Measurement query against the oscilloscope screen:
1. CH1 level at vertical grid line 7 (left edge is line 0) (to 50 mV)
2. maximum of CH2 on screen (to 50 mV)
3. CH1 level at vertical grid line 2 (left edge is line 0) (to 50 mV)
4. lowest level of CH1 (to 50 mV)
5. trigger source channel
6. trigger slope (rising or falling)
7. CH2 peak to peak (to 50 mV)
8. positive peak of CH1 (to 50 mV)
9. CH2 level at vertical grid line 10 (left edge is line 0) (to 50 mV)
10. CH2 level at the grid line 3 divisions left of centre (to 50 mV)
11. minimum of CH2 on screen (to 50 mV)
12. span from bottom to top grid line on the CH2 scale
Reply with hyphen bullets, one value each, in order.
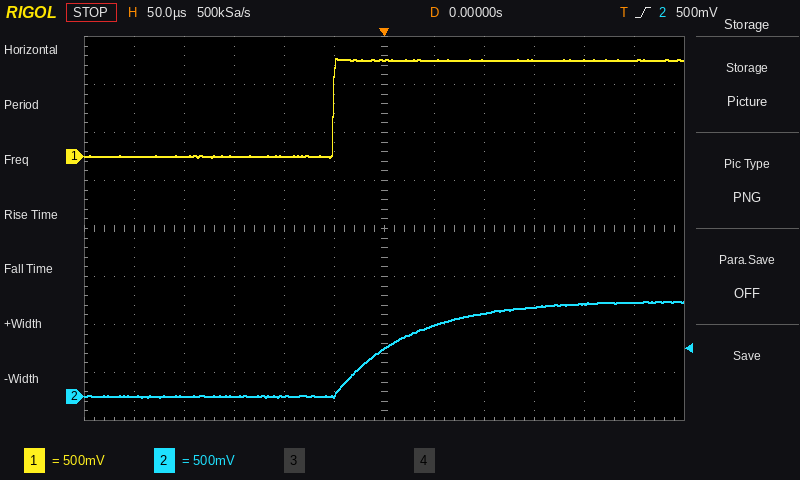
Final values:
- 1.00 V
- 1.00 V
- 0 mV
- 0 mV
- CH2
- rising
- 1.00 V
- 1.00 V
- 950 mV
- 0 mV
- 0 mV
- 4 V
